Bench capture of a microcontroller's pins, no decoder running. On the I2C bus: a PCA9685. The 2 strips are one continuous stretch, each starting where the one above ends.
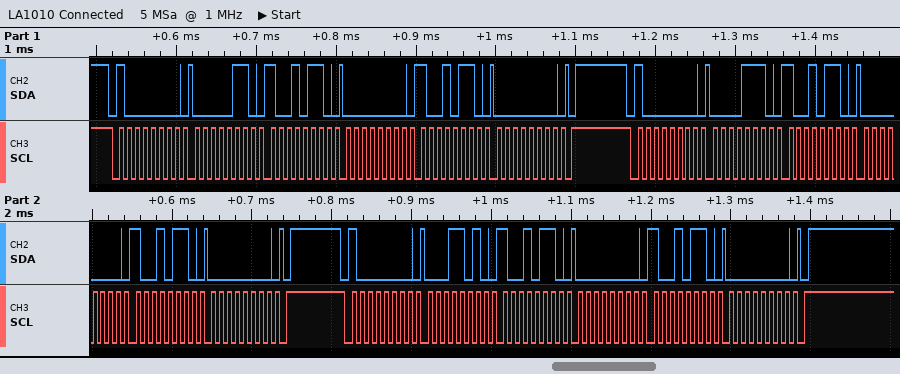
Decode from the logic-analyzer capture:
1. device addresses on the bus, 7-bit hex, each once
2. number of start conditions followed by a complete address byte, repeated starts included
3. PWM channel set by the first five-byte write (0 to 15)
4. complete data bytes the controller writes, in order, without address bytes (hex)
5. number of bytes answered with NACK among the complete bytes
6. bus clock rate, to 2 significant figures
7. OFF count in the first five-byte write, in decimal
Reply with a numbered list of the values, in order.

1. 0x40
2. 3
3. 0
4. 06 96 00 96 00 0E 96 00 96 00 1A 96 00 96 00
5. 0
6. 100 kHz
7. 150
